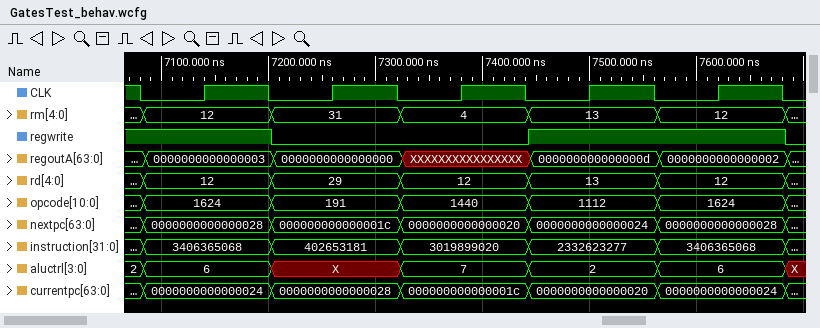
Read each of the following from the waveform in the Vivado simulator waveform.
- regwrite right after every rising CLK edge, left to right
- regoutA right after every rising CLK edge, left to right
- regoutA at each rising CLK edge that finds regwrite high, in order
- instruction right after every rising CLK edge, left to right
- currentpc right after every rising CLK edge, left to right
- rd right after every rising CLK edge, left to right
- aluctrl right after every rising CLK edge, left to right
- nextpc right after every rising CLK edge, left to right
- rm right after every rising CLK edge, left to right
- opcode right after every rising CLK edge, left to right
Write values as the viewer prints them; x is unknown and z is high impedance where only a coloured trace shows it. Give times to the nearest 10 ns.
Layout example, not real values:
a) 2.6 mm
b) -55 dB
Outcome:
a) 1 0 0 1 1
b) 0000000000000003, 0000000000000000, XXXXXXXXXXXXXXXX, 000000000000000d, 0000000000000002
c) 0000000000000003, 000000000000000d, 0000000000000002
d) 3406365068, 402653181, 3019899020, 2332623277, 3406365068
e) 0000000000000024, 0000000000000028, 000000000000001c, 0000000000000020, 0000000000000024
f) 12, 29, 12, 13, 12
g) 6, X, 7, 2, 6
h) 0000000000000028, 000000000000001c, 0000000000000020, 0000000000000024, 0000000000000028
i) 12, 31, 4, 13, 12
j) 1624, 191, 1440, 1112, 1624
